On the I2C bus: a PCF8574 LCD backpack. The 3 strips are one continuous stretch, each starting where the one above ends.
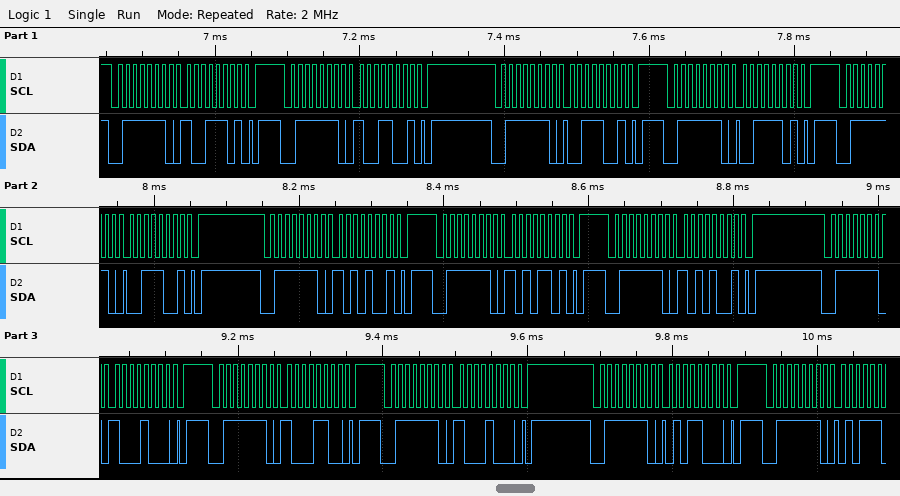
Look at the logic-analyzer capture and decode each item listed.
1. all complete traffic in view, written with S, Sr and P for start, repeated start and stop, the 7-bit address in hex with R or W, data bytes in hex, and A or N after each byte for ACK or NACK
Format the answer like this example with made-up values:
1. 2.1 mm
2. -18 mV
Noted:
1. S 3FW A 9D A P S 3FW A 99 A P S 3FW A 39 A P S 3FW A 3D A P S 3FW A 39 A P S 3FW A A9 A P S 3FW A AD A P S 3FW A A9 A P S 3FW A 88 A P S 3FW A 8C A P S 3FW A 88 A P S 3FW A 58 A P S 3FW A
